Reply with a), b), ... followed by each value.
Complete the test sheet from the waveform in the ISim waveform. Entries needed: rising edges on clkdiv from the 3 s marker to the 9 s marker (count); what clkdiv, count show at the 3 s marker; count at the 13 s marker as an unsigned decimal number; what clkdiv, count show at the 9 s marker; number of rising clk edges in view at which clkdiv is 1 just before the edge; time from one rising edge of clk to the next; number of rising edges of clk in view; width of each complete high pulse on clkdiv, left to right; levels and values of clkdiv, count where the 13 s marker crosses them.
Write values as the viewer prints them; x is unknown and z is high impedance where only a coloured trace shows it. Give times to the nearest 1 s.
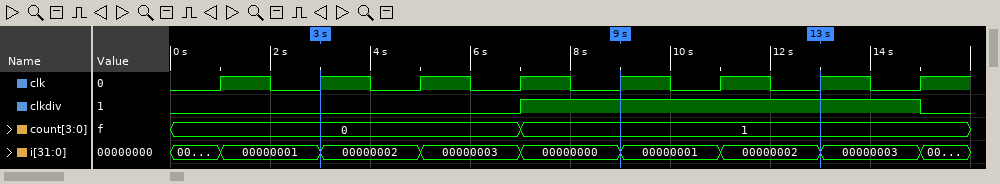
a) 1
b) clkdiv=0, count=0
c) 1
d) clkdiv=1, count=1
e) 4
f) 2 s
g) 8
h) 8 s
i) clkdiv=1, count=1
